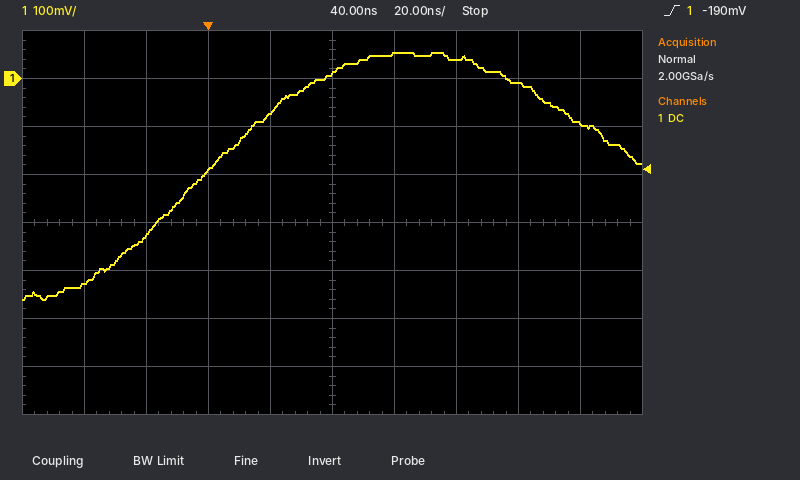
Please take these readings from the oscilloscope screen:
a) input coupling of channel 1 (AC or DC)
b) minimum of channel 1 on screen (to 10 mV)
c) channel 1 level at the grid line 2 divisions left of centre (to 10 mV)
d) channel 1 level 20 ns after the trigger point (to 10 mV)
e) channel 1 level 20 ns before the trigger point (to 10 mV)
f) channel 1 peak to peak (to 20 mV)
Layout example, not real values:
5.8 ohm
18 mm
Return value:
DC
-460 mV
-190 mV
-70 mV
-330 mV
520 mV
